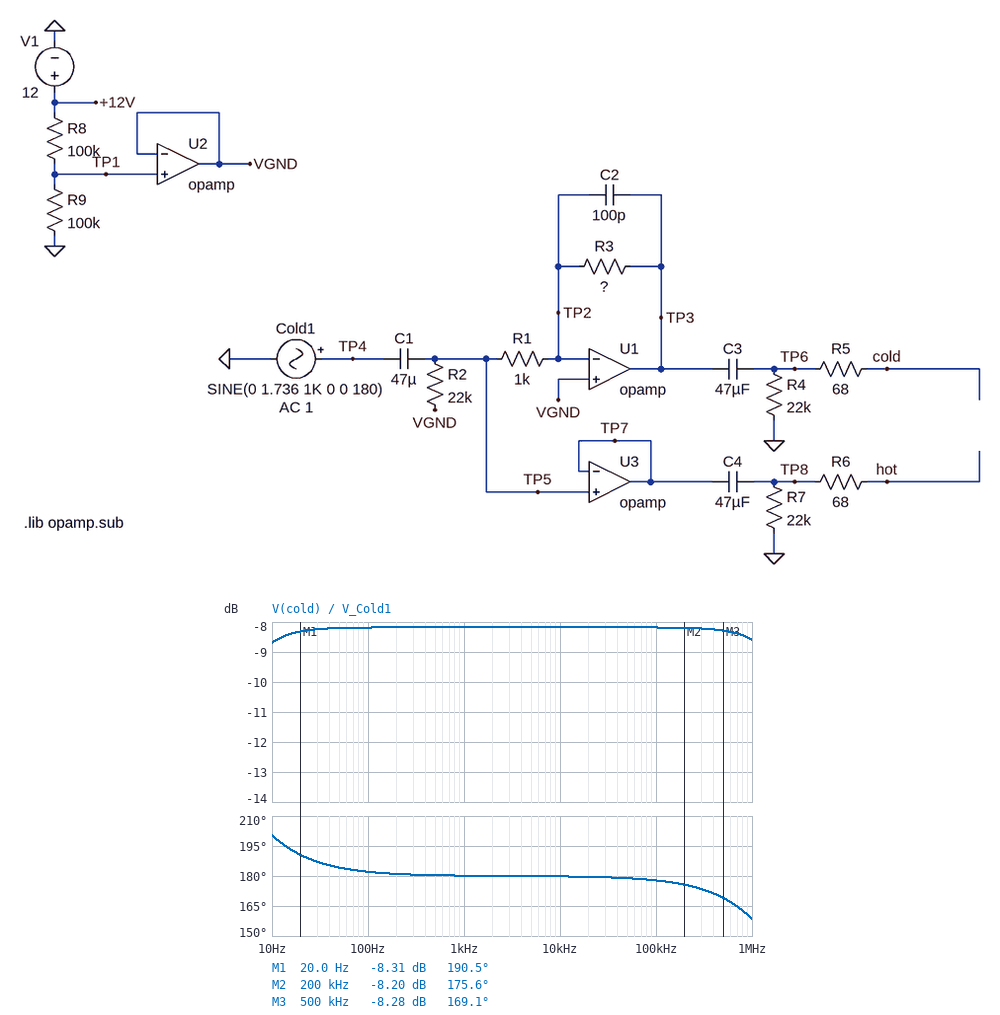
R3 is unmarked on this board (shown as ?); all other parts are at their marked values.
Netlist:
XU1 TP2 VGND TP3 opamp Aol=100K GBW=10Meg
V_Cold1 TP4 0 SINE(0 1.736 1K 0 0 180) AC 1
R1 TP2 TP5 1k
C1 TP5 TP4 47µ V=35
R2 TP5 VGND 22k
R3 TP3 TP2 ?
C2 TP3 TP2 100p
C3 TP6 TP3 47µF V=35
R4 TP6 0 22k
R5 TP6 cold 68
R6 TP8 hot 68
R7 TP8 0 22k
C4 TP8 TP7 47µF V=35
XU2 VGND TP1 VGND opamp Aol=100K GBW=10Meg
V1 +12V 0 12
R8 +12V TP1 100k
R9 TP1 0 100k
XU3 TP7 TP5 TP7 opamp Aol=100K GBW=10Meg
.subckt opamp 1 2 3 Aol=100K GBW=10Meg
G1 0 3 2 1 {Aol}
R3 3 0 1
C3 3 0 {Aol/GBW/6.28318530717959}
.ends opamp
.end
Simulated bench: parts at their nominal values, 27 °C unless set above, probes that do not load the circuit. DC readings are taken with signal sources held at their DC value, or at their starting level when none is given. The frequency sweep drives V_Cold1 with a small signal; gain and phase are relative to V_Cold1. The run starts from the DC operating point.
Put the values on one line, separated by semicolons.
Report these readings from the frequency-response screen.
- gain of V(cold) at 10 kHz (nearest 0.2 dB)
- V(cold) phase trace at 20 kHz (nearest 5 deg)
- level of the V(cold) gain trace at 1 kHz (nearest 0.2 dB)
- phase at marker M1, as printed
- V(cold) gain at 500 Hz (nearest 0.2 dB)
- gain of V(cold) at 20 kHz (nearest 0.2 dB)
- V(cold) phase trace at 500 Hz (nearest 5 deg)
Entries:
-8.2 dB; 180 deg; -8.2 dB; 190.5 deg; -8.2 dB; -8.2 dB; 180 deg
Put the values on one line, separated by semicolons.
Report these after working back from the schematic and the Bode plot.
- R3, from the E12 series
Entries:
390 Ω
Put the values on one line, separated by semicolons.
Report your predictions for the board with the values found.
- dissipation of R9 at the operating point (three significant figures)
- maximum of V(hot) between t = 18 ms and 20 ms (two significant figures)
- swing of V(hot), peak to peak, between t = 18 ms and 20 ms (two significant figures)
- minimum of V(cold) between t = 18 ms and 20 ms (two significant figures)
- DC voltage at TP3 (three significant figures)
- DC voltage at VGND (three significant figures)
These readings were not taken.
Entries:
360 µW; 1.7 V; 3.5 V; -680 mV; 6.00 V; 6.00 V
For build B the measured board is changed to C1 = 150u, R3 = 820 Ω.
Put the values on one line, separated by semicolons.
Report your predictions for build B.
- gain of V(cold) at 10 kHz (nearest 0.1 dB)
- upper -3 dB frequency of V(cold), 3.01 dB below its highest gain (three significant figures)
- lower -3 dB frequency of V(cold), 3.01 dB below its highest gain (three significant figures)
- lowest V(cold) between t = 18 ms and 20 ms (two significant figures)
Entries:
-1.7 dB; 1.60 MHz; 1.13 Hz; -1.4 V
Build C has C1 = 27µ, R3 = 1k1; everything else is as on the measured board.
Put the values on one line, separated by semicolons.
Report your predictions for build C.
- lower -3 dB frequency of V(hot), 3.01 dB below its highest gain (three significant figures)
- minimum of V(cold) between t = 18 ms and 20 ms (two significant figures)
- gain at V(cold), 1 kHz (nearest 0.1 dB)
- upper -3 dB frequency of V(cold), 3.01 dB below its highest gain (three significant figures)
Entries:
6.17 Hz; -1.9 V; 0.8 dB; 1.21 MHz
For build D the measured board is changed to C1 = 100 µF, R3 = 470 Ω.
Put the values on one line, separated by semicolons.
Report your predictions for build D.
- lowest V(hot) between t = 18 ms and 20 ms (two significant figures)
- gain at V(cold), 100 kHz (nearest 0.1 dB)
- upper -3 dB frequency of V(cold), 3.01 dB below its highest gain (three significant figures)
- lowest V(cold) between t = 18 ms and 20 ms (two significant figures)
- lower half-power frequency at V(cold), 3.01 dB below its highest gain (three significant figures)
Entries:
-1.7 V; -6.6 dB; 2.65 MHz; -820 mV; 1.68 Hz
